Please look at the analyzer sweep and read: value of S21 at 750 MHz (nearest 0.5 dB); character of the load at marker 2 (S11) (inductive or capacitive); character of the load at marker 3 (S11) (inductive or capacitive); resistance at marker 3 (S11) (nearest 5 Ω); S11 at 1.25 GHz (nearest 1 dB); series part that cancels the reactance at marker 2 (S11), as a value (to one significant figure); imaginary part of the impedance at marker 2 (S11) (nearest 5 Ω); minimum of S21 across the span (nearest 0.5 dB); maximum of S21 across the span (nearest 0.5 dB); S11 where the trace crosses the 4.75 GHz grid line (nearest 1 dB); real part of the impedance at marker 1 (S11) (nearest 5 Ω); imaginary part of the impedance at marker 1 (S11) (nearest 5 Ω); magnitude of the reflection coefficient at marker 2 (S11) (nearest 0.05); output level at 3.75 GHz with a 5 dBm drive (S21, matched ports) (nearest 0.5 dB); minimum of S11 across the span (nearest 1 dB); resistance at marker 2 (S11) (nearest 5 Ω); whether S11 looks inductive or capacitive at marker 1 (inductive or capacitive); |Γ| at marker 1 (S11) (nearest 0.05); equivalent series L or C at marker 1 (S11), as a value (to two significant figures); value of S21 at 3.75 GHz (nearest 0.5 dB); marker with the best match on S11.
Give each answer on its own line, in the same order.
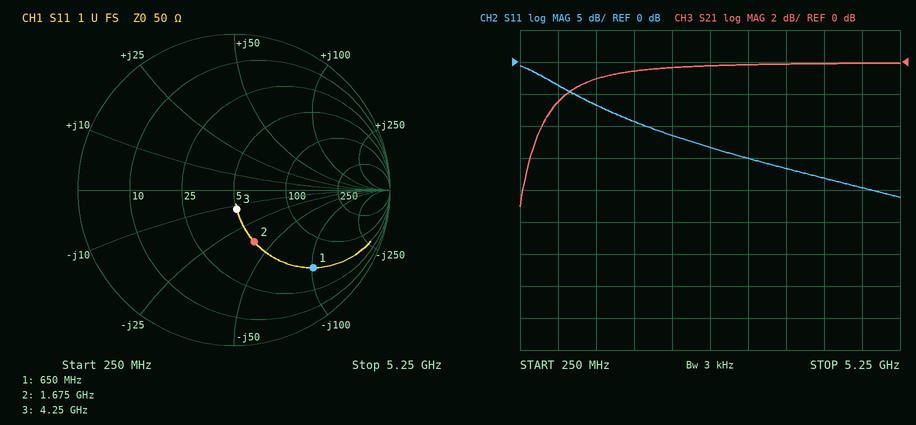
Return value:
-2.5 dB
capacitive
capacitive
50 Ω
-7 dB
4 nH
-40 Ω
-9.0 dB
0.0 dB
-20 dB
50 Ω
-100 Ω
0.35
5.0 dBm
-21 dB
50 Ω
capacitive
0.70
2.4 pF
0.0 dB
marker 3
